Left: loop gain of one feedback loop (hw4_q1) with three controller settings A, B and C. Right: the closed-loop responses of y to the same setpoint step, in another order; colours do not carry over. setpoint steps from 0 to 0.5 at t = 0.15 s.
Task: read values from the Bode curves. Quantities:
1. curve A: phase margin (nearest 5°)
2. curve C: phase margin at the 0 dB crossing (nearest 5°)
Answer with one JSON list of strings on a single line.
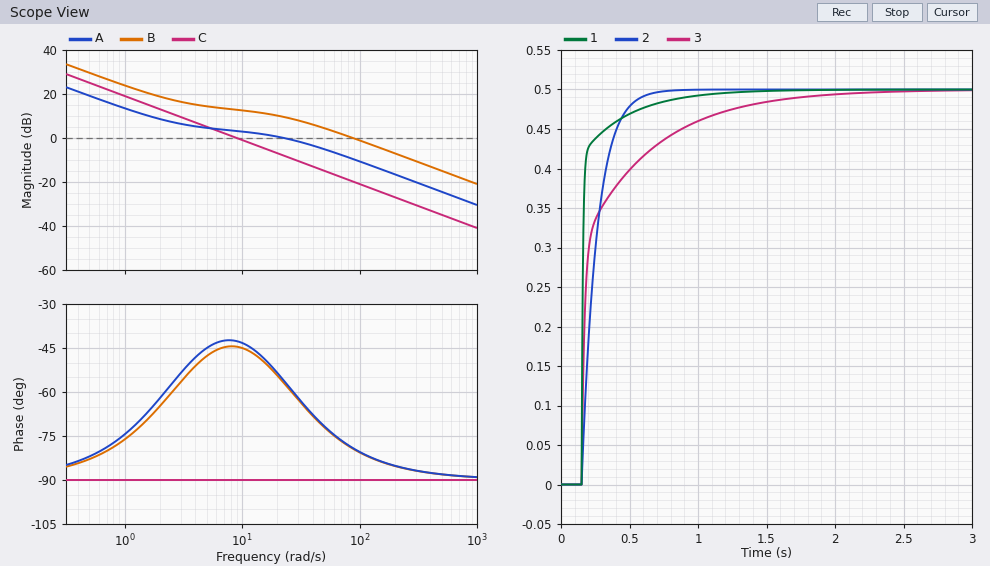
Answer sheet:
["125°", "90°"]
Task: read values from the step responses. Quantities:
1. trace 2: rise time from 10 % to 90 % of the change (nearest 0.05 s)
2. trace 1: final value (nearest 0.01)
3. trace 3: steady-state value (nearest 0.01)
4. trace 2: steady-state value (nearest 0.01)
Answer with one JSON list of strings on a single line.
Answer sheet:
["0.25 s", "0.50", "0.50", "0.50"]
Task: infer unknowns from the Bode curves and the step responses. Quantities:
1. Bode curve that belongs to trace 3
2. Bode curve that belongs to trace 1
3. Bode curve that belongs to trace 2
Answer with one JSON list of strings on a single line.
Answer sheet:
["A", "B", "C"]
